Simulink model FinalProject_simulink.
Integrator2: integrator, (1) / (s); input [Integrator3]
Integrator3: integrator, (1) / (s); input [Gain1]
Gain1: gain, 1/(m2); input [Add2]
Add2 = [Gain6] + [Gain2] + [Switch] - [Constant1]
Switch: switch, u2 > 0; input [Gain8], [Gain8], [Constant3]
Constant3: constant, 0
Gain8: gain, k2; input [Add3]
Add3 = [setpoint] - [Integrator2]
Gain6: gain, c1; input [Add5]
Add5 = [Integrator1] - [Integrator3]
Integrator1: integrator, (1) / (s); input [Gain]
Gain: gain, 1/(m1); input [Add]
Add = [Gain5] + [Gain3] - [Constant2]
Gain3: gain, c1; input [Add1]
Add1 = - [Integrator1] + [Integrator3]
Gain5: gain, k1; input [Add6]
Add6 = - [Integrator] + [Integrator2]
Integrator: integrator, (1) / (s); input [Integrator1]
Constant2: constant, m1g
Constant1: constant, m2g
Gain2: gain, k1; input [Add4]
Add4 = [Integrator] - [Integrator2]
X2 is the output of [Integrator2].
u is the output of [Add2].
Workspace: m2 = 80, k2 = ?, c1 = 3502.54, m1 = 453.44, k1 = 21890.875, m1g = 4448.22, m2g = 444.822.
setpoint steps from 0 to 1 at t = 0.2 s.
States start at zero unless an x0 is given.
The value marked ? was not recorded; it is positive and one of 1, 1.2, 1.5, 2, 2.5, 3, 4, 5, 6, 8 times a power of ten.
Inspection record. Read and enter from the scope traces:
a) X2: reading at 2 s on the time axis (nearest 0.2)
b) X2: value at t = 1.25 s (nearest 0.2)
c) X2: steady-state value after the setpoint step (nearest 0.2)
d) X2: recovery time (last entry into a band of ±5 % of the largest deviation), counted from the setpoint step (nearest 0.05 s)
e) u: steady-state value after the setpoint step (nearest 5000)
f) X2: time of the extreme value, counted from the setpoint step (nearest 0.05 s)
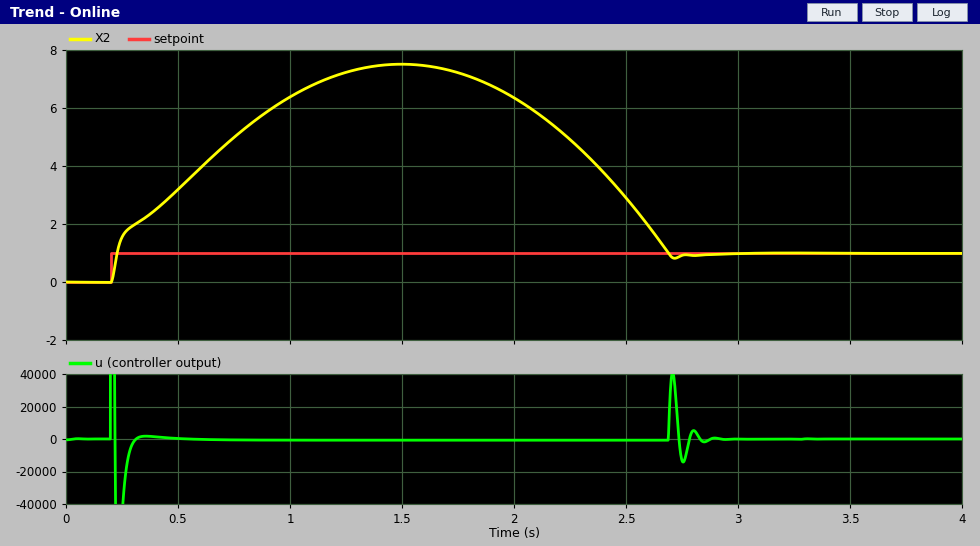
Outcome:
6.4
7.2
1.0
2.45 s
0
1.30 s
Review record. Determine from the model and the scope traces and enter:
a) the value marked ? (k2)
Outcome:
400000
